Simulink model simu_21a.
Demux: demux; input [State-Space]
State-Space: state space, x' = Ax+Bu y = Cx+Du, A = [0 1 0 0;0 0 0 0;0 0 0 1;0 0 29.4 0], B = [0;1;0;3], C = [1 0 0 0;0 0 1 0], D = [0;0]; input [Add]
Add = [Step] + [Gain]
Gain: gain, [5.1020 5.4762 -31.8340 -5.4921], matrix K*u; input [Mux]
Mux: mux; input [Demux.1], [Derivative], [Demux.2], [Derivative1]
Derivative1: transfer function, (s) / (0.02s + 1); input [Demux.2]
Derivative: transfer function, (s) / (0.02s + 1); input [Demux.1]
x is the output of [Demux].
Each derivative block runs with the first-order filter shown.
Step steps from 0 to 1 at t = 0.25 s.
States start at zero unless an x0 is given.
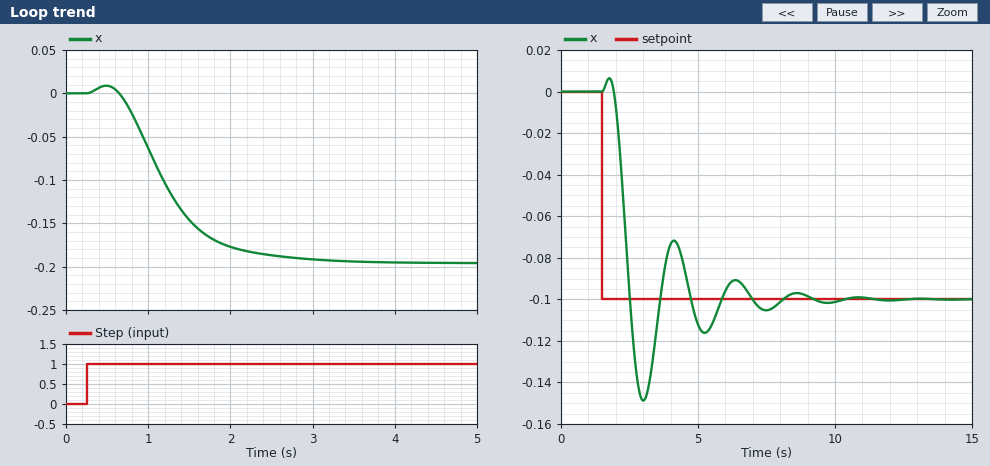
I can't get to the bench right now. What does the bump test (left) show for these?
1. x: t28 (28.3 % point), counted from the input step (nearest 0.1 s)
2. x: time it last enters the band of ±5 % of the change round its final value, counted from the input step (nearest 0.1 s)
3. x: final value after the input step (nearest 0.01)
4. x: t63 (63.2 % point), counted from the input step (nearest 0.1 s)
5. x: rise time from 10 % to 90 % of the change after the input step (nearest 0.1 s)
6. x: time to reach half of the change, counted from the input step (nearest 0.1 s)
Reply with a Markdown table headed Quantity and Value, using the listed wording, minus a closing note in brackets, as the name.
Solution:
| Quantity | Value |
|---|---|
| x: t28 (28.3 % point), counted from the input step | 0.7 s |
| x: time it last enters the band of ±5 % of the change round its final value, counted from the input step | 2.2 s |
| x: final value after the input step | -0.20 |
| x: t63 (63.2 % point), counted from the input step | 1.1 s |
| x: rise time from 10 % to 90 % of the change after the input step | 1.2 s |
| x: time to reach half of the change, counted from the input step | 0.9 s |
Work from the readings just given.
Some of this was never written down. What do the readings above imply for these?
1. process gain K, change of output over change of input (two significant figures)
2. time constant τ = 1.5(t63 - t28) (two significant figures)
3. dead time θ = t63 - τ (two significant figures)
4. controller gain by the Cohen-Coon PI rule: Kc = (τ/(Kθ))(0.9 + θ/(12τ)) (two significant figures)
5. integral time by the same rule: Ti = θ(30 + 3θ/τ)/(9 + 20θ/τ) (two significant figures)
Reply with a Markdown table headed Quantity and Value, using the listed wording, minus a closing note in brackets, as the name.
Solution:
| Quantity | Value |
|---|---|
| process gain K, change of output over change of input | -0.20 |
| time constant τ = 1.5(t63 - t28) | 0.60 s |
| dead time θ = t63 - τ | 0.50 s |
| controller gain by the Cohen-Coon PI rule: Kc = (τ/(Kθ))(0.9 + θ/(12τ)) | -5.8 |
| integral time by the same rule: Ti = θ(30 + 3θ/τ)/(9 + 20θ/τ) | 0.63 s |
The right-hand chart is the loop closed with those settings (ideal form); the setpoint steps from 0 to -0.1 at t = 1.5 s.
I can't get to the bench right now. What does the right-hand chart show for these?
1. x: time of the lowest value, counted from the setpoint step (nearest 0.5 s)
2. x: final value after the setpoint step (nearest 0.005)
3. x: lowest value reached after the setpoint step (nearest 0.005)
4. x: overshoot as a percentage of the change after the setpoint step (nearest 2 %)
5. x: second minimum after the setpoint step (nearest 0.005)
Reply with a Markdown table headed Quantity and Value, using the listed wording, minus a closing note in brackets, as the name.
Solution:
| Quantity | Value |
|---|---|
| x: time of the lowest value, counted from the setpoint step | 1.5 s |
| x: final value after the setpoint step | -0.100 |
| x: lowest value reached after the setpoint step | -0.150 |
| x: overshoot as a percentage of the change after the setpoint step | 48 % |
| x: second minimum after the setpoint step | -0.115 |
